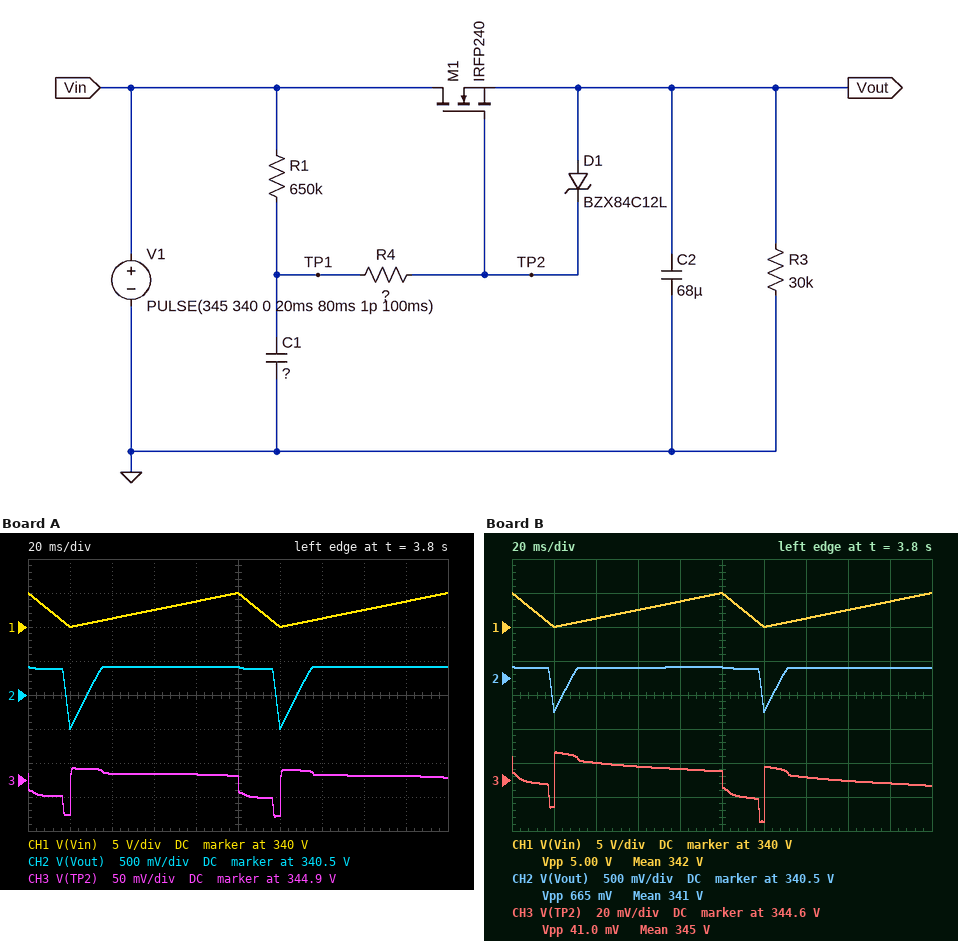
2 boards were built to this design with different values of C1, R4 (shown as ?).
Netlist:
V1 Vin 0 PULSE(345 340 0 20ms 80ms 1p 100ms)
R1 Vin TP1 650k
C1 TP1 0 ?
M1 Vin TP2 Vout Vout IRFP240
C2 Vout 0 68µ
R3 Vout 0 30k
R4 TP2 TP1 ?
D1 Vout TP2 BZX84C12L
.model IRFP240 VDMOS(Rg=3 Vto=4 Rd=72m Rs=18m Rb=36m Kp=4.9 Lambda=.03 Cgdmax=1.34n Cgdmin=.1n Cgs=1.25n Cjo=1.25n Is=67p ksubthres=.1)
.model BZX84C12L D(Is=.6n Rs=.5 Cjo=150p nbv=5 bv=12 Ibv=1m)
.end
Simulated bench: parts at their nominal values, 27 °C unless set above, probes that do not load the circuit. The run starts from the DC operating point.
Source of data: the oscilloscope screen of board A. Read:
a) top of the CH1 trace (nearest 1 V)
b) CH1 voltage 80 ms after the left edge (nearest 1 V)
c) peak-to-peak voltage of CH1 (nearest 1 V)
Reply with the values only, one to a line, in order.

345 V
344 V
5 V
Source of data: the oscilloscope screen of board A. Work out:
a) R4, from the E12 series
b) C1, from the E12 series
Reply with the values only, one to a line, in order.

82 kΩ
150 µF
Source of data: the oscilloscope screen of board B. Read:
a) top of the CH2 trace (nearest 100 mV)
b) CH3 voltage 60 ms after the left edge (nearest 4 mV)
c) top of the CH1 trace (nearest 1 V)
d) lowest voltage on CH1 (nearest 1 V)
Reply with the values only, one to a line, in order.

340.7 V
344.648 V
345 V
340 V
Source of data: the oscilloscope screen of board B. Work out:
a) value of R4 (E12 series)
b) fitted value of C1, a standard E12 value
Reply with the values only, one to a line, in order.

39 kΩ
39 µF
